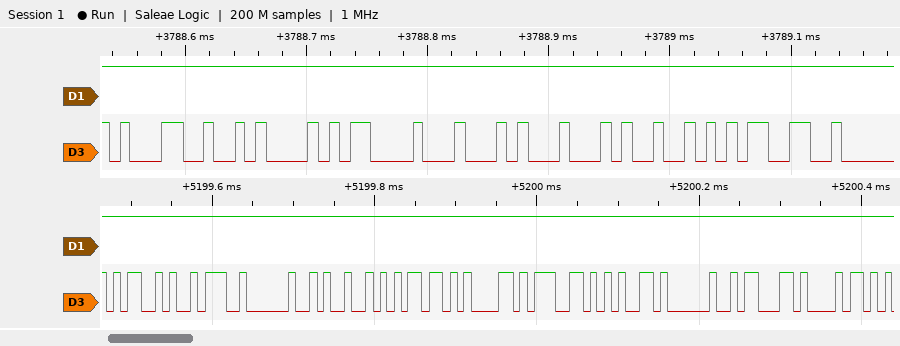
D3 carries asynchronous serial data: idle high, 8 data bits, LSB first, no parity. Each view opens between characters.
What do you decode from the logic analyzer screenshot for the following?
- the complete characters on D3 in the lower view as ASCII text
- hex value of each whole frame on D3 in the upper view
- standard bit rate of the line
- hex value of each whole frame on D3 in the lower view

"M: Image ch"
31, 0A, 0D, 44, 44, 52, 33
115200 baud
4D, 3A, 20, 49, 6D, 61, 67, 65, 20, 63, 68
